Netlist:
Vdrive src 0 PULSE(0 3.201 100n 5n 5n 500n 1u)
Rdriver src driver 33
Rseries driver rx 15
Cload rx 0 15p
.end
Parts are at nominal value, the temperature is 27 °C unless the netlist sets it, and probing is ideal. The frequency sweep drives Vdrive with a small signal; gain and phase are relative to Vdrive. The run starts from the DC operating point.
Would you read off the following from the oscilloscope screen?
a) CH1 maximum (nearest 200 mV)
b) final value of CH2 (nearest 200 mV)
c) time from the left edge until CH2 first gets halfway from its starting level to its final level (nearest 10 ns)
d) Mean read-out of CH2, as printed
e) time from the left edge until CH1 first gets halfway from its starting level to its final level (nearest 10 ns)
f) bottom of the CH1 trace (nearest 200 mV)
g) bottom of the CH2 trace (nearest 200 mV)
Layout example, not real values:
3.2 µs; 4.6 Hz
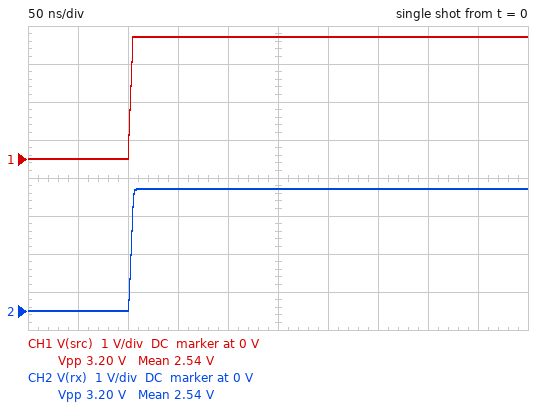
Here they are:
3.2 V; 3.2 V; 100 ns; 2.54 V; 100 ns; 0 V; 0 V
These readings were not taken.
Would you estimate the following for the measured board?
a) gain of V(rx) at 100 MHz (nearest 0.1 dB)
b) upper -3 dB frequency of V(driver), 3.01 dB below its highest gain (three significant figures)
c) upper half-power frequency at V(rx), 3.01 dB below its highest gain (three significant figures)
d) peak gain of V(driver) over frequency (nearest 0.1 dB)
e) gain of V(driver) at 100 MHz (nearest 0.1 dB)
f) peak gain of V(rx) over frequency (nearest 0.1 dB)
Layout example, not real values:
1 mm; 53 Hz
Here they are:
-0.8 dB; 246 MHz; 221 MHz; 0 dB; -0.7 dB; 0 dB
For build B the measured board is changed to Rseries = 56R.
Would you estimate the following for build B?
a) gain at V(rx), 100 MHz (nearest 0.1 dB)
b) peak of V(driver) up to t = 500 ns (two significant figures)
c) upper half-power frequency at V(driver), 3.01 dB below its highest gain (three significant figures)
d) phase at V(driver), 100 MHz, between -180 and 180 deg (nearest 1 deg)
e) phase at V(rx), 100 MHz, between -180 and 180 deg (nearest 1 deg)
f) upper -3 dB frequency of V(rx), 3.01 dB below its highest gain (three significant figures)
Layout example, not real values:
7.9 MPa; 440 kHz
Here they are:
-2.3 dB; 3.2 V; 261 MHz; -12 deg; -40 deg; 119 MHz
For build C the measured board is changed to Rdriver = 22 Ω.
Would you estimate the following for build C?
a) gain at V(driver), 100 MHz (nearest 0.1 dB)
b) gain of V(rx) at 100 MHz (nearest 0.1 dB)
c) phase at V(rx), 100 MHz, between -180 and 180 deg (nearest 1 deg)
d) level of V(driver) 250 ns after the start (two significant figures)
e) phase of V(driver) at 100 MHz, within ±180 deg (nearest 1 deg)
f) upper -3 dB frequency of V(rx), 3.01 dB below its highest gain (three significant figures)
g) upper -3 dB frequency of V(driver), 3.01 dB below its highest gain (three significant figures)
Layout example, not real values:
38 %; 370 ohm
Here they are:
-0.4 dB; -0.5 dB; -19 deg; 3.2 V; -11 deg; 287 MHz; 350 MHz
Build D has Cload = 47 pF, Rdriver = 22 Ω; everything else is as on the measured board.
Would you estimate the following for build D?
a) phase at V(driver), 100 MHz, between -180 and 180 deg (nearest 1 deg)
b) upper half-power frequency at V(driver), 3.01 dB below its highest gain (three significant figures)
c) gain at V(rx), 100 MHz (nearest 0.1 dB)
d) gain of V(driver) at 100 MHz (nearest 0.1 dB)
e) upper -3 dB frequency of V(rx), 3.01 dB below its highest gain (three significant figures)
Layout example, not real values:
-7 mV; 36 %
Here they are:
-24 deg; 112 MHz; -3.4 dB; -2.6 dB; 91.5 MHz
